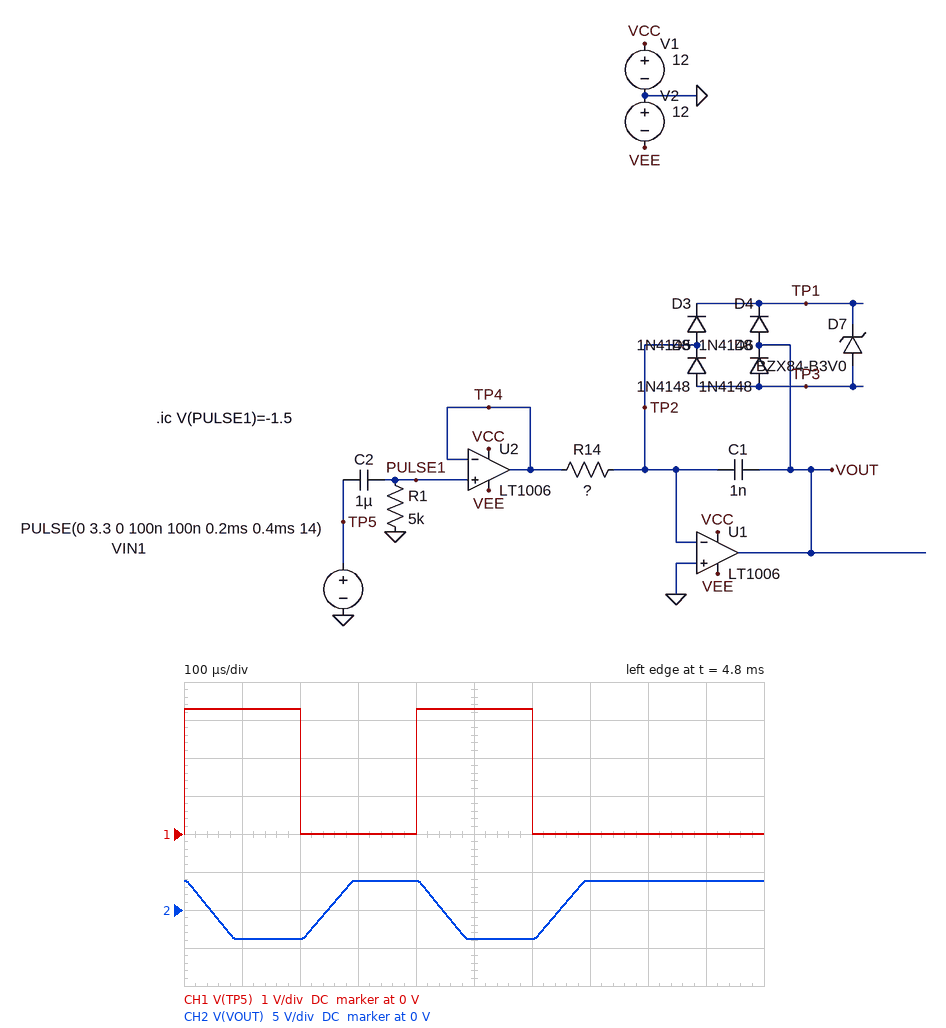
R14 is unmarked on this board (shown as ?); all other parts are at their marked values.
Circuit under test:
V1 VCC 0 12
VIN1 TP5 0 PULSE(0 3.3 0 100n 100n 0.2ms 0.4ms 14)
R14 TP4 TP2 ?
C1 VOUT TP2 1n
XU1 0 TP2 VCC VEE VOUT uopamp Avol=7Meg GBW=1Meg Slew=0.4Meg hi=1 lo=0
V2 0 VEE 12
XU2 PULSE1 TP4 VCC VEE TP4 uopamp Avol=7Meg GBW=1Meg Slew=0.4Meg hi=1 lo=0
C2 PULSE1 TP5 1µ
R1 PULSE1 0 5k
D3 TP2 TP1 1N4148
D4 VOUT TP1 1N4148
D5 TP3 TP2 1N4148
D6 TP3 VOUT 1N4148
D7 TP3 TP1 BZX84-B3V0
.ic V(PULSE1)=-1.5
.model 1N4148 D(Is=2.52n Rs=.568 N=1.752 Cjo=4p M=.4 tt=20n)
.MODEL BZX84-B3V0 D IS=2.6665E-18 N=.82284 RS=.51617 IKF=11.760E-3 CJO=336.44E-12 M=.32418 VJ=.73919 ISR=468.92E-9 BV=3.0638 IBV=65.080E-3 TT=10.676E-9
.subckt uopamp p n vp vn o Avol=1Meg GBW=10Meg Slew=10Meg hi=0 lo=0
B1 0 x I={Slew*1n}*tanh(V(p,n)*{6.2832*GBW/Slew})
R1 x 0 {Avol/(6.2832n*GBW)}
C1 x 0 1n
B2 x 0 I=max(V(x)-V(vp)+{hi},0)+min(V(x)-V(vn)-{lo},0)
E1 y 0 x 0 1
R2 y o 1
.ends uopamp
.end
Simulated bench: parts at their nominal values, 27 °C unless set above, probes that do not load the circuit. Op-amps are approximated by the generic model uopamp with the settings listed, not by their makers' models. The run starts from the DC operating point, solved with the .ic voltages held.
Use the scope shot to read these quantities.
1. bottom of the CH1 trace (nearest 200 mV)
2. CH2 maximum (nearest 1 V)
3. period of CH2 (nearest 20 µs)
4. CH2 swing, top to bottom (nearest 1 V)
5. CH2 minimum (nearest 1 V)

0 V
4 V
400 µs
8 V
-4 V
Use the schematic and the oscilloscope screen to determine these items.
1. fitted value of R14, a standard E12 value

18 kΩ
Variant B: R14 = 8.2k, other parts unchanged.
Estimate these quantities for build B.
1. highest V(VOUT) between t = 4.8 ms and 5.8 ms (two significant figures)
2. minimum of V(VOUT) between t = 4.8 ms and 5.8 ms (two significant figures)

4.0 V
-4.0 V
